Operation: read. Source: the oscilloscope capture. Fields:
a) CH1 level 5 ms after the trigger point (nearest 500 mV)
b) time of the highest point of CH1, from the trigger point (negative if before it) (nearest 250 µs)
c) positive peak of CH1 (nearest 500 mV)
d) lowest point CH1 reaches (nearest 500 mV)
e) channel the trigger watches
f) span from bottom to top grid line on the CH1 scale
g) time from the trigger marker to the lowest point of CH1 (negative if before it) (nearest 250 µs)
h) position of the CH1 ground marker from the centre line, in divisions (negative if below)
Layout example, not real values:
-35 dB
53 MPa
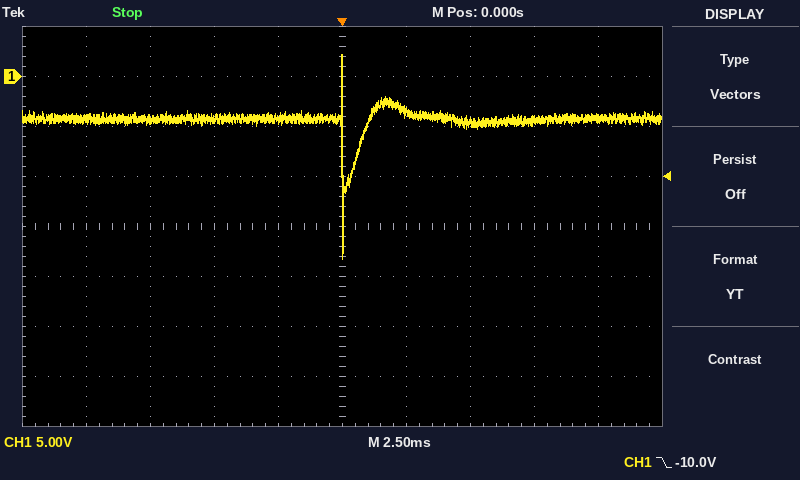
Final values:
-4.5 V
0.00 ms
2.0 V
-18.0 V
CH1
40 V
0.00 ms
+3.0 div
